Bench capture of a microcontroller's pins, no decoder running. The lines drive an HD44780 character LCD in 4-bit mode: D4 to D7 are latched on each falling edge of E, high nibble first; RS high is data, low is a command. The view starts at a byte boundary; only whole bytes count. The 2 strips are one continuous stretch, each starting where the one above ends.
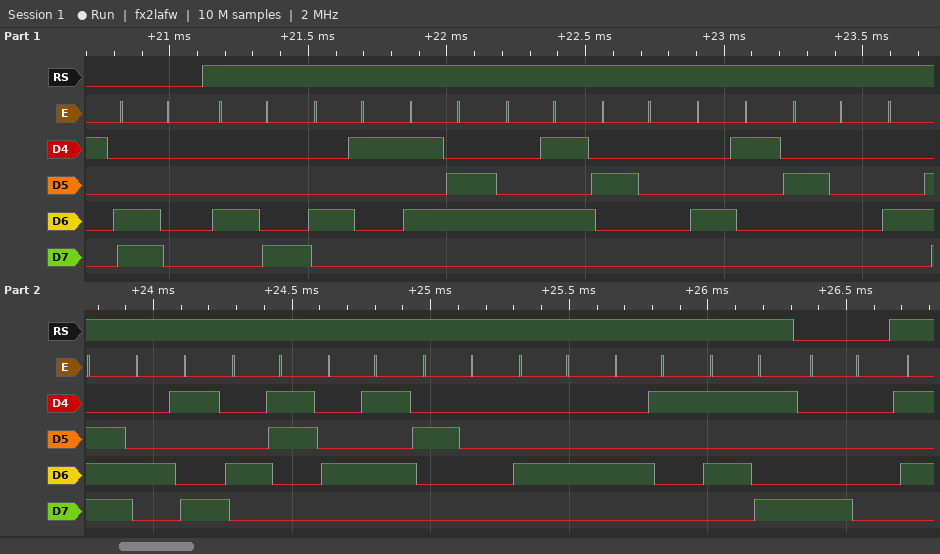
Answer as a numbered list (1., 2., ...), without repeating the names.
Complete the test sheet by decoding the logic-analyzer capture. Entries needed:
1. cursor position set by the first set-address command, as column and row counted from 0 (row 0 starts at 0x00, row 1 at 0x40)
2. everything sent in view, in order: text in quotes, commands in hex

1. column 0, row 1
2. 0xC0 "HAVE A NICE DAY" 0x80
